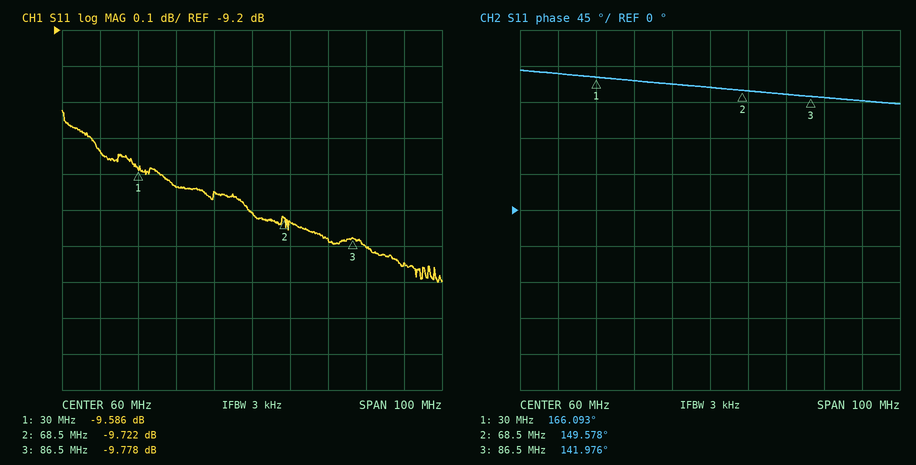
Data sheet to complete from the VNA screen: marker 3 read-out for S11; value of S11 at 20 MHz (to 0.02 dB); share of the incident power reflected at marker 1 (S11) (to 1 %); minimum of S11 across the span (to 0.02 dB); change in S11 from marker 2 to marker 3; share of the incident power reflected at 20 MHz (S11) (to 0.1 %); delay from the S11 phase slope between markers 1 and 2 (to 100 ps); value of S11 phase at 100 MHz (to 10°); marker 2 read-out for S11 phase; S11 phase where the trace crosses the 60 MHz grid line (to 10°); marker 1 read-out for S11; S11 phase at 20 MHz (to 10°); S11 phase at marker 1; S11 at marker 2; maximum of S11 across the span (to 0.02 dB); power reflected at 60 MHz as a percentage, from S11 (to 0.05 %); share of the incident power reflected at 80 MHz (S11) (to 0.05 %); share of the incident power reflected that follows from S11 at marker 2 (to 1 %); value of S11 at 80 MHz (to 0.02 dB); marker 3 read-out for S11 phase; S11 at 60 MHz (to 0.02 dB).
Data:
-9.778 dB
-9.54 dB
11 %
-9.90 dB
-0.056 dB
11.1 %
1.2 ns
140°
149.578°
150°
-9.586 dB
170°
166.093°
-9.722 dB
-9.42 dB
10.70 %
10.50 %
11 %
-9.78 dB
141.976°
-9.70 dB
